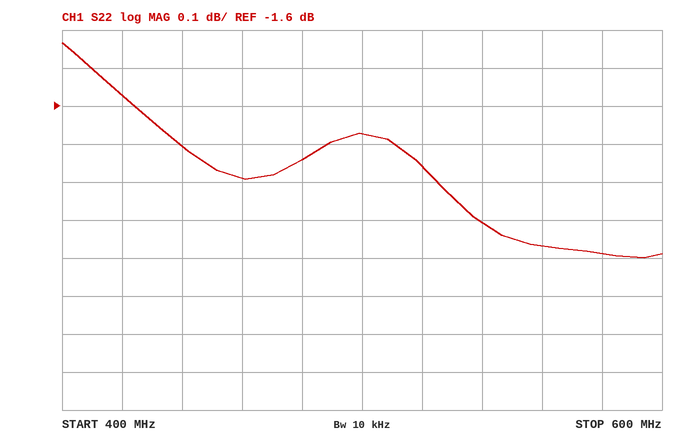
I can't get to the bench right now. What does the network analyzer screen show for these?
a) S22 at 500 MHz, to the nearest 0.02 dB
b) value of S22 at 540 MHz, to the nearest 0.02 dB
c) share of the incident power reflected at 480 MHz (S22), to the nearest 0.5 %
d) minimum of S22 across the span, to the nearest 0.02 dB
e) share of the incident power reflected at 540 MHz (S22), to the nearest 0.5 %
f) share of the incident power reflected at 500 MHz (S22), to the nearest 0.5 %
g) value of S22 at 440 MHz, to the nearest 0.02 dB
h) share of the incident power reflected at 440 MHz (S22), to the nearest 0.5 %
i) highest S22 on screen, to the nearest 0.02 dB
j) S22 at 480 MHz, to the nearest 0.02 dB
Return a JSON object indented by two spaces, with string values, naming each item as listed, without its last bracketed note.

{
  "S22 at 500 MHz, to the nearest 0.02 dB": "-1.68 dB",
  "value of S22 at 540 MHz, to the nearest 0.02 dB": "-1.90 dB",
  "share of the incident power reflected at 480 MHz (S22), to the nearest 0.5 %": "67.0 %",
  "minimum of S22 across the span, to the nearest 0.02 dB": "-2.00 dB",
  "share of the incident power reflected at 540 MHz (S22), to the nearest 0.5 %": "64.5 %",
  "share of the incident power reflected at 500 MHz (S22), to the nearest 0.5 %": "68.0 %",
  "value of S22 at 440 MHz, to the nearest 0.02 dB": "-1.70 dB",
  "share of the incident power reflected at 440 MHz (S22), to the nearest 0.5 %": "67.5 %",
  "highest S22 on screen, to the nearest 0.02 dB": "-1.44 dB",
  "S22 at 480 MHz, to the nearest 0.02 dB": "-1.74 dB"
}
